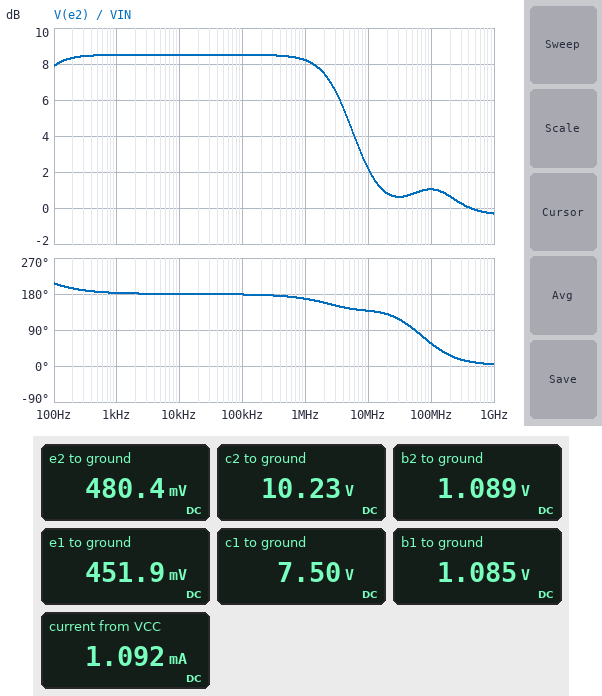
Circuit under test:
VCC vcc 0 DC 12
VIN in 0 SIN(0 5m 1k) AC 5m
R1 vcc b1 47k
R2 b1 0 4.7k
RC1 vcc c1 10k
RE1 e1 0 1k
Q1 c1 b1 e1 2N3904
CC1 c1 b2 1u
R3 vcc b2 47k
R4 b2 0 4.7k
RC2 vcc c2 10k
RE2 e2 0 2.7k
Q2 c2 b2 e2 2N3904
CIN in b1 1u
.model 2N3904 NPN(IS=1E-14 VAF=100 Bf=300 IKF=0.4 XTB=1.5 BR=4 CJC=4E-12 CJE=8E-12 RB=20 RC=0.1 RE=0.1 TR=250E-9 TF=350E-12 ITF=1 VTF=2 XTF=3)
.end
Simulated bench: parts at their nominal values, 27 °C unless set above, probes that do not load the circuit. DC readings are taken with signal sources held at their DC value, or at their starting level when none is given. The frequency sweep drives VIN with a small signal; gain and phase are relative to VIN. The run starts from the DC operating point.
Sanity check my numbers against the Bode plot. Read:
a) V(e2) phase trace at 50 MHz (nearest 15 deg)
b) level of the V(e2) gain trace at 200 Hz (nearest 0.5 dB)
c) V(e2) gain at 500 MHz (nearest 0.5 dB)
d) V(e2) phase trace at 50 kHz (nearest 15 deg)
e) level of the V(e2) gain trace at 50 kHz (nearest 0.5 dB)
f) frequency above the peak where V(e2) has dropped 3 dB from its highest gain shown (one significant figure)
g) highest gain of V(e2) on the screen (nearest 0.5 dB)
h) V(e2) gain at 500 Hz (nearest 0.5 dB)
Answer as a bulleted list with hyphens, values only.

- 90 deg
- 8.5 dB
- 0 dB
- 180 deg
- 8.5 dB
- 4 MHz
- 8.5 dB
- 8.5 dB
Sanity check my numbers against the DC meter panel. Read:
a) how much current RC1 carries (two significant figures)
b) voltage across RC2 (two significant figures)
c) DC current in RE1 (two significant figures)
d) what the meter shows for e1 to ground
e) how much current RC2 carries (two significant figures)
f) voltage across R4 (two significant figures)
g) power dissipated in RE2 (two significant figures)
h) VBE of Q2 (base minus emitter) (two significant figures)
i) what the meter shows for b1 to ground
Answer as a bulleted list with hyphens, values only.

- 450 µA
- 1.8 V
- 450 µA
- 451.9 mV
- 180 µA
- 1.1 V
- 85 µW
- 610 mV
- 1.085 V
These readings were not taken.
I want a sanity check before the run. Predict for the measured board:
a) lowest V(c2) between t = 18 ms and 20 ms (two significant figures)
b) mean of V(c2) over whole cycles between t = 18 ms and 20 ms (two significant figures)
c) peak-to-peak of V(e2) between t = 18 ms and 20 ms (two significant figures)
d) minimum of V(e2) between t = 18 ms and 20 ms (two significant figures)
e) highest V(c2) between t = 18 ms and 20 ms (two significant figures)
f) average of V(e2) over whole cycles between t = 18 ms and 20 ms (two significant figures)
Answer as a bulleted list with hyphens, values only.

- 10 V
- 10 V
- 27 mV
- 470 mV
- 10 V
- 480 mV
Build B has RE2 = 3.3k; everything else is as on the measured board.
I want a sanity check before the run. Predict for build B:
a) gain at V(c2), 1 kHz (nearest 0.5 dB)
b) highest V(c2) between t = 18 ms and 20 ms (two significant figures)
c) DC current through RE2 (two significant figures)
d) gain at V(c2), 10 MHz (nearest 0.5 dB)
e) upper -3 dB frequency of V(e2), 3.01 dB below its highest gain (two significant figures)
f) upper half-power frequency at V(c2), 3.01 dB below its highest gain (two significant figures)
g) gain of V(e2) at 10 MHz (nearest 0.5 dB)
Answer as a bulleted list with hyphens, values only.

- 18.0 dB
- 11 V
- 150 µA
- 10.0 dB
- 4.6 MHz
- 3.9 MHz
- 3.0 dB
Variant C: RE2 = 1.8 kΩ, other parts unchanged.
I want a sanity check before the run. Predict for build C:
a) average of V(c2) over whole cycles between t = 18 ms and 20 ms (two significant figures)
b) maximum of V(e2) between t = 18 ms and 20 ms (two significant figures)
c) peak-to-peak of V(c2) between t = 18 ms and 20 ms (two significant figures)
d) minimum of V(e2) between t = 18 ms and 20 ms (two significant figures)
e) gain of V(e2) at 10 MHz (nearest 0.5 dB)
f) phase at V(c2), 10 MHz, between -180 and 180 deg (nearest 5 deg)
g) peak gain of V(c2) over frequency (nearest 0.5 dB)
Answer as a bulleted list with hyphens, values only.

- 9.4 V
- 480 mV
- 150 mV
- 460 mV
- 0.5 dB
- -110 deg
- 23.5 dB
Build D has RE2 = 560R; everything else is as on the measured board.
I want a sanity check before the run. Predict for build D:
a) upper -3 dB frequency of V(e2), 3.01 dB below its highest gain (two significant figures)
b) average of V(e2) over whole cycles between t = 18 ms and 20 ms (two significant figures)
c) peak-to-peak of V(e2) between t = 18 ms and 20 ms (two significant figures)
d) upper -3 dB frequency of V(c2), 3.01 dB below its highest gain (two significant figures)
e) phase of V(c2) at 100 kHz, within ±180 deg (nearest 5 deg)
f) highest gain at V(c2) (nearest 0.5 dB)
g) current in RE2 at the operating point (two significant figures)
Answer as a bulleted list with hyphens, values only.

- 1.1 MHz
- 430 mV
- 26 mV
- 1.0 MHz
- -5 deg
- 33.5 dB
- 770 µA
